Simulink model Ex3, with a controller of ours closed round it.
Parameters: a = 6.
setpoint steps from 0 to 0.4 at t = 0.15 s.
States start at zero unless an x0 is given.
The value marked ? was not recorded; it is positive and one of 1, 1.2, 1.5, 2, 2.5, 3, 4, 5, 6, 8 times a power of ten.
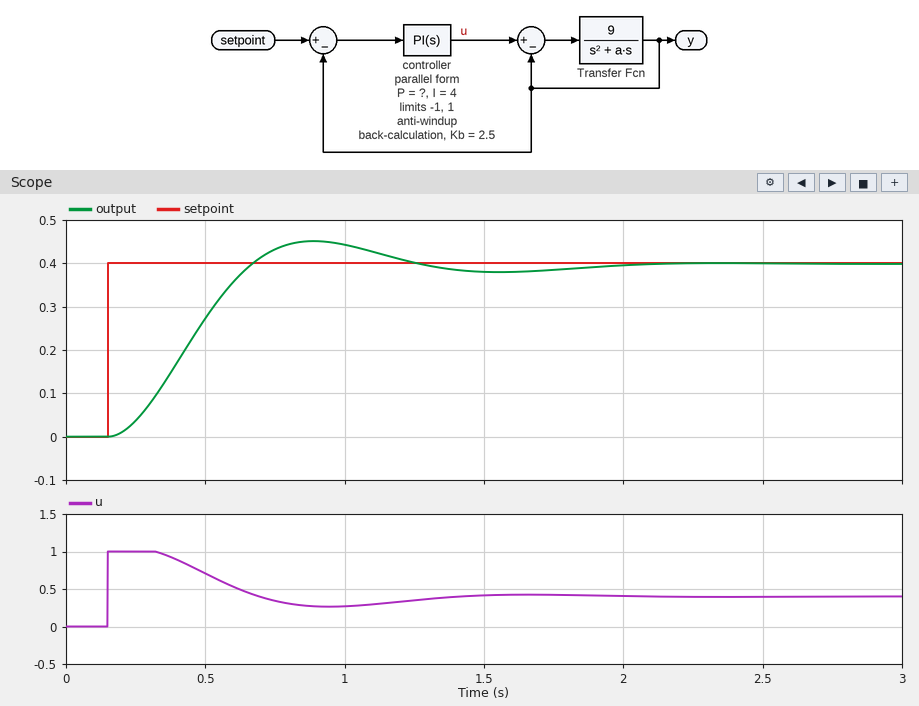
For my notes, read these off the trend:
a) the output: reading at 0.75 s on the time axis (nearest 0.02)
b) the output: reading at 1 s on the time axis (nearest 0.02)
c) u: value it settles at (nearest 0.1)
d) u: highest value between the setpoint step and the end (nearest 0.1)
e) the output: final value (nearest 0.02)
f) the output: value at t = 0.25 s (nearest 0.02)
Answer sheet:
0.44
0.44
0.4
1.0
0.40
0.04
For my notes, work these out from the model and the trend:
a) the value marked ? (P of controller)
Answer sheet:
2.5
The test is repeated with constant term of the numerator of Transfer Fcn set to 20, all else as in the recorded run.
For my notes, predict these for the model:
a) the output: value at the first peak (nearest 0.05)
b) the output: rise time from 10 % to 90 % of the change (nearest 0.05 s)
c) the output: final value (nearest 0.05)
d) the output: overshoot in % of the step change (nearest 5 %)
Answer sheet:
0.45
0.20 s
0.40
15 %
